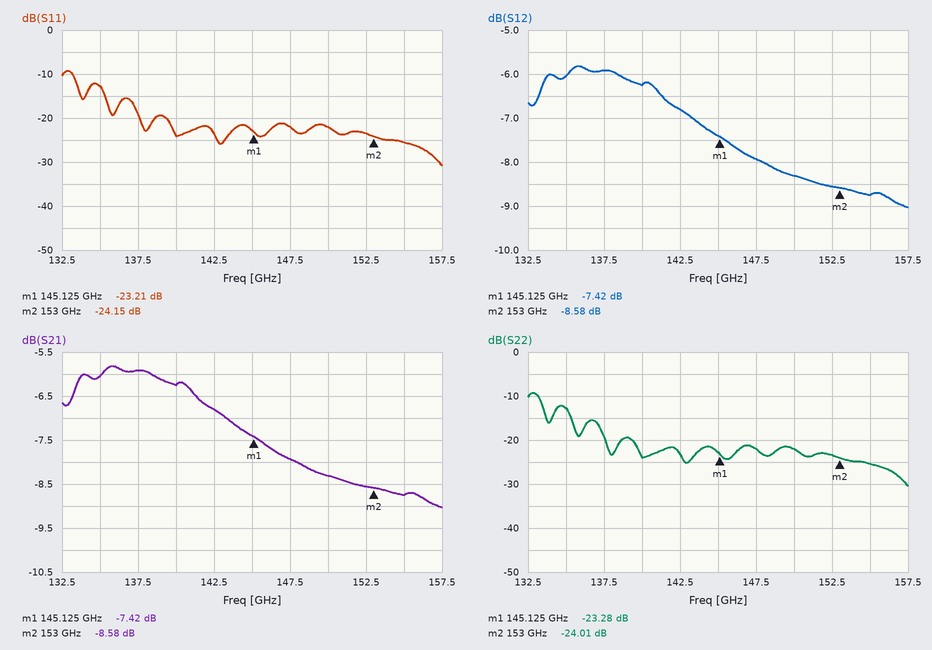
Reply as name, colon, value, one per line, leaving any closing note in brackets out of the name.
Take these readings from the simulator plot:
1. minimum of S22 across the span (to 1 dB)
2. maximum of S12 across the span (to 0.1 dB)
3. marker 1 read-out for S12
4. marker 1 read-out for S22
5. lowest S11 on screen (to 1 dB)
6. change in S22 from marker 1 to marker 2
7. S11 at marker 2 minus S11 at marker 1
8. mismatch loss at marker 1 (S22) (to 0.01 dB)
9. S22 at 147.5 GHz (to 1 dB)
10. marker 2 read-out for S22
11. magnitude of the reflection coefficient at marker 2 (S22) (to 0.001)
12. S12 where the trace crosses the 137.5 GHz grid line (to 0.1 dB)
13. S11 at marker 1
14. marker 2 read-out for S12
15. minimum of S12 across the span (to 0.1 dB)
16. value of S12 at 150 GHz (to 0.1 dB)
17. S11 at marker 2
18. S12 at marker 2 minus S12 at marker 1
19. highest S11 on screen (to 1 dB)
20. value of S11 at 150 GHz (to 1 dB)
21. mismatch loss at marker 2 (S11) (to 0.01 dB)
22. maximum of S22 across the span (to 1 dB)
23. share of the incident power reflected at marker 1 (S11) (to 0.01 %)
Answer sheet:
minimum of S22 across the span: -30 dB
maximum of S12 across the span: -5.8 dB
marker 1 read-out for S12: -7.42 dB
marker 1 read-out for S22: -23.28 dB
lowest S11 on screen: -31 dB
change in S22 from marker 1 to marker 2: -0.73 dB
S11 at marker 2 minus S11 at marker 1: -0.94 dB
mismatch loss at marker 1 (S22): 0.02 dB
S22 at 147.5 GHz: -22 dB
marker 2 read-out for S22: -24.01 dB
magnitude of the reflection coefficient at marker 2 (S22): 0.063
S12 where the trace crosses the 137.5 GHz grid line: -5.9 dB
S11 at marker 1: -23.21 dB
marker 2 read-out for S12: -8.58 dB
minimum of S12 across the span: -9.0 dB
value of S12 at 150 GHz: -8.3 dB
S11 at marker 2: -24.15 dB
S12 at marker 2 minus S12 at marker 1: -1.16 dB
highest S11 on screen: -9 dB
value of S11 at 150 GHz: -22 dB
mismatch loss at marker 2 (S11): 0.02 dB
maximum of S22 across the span: -9 dB
share of the incident power reflected at marker 1 (S11): 0.48 %
